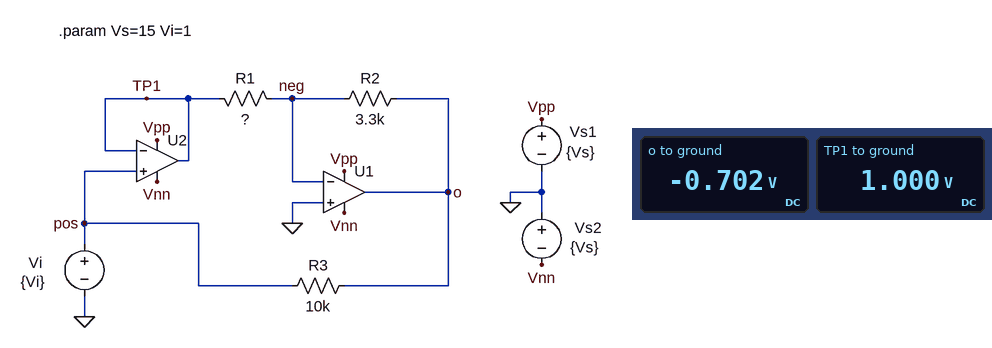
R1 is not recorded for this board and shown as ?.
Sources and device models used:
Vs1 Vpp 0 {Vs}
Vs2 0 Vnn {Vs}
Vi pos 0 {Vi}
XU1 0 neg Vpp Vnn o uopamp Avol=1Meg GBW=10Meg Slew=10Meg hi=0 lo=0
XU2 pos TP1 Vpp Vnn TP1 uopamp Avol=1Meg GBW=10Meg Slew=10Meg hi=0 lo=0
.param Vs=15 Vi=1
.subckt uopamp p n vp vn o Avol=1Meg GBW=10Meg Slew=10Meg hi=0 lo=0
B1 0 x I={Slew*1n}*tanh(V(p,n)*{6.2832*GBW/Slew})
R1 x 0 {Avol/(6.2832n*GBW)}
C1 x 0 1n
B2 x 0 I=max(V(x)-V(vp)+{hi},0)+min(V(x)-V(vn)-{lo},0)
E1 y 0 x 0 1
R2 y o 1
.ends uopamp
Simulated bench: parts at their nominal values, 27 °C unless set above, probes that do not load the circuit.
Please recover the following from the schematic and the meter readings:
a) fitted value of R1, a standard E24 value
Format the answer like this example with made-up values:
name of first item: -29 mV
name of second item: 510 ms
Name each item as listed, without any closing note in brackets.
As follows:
fitted value of R1, a standard E24 value: 4.7 kΩ
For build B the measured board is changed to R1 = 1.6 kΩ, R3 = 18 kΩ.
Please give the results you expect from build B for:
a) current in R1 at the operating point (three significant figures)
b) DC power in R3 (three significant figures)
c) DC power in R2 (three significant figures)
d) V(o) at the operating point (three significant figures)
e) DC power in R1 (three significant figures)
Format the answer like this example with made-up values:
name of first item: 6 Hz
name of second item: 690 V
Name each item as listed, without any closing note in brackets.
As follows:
current in R1 at the operating point: 625 µA
DC power in R3: 521 µW
DC power in R2: 1.29 mW
V(o) at the operating point: -2.06 V
DC power in R1: 625 µW
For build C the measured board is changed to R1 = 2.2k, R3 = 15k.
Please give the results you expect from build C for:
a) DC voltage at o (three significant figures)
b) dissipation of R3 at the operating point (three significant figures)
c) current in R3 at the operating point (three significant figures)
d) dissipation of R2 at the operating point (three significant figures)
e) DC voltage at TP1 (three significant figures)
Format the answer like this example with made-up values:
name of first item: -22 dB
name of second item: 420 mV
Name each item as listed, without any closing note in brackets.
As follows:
DC voltage at o: -1.50 V
dissipation of R3 at the operating point: 417 µW
current in R3 at the operating point: 167 µA
dissipation of R2 at the operating point: 682 µW
DC voltage at TP1: 1.00 V
